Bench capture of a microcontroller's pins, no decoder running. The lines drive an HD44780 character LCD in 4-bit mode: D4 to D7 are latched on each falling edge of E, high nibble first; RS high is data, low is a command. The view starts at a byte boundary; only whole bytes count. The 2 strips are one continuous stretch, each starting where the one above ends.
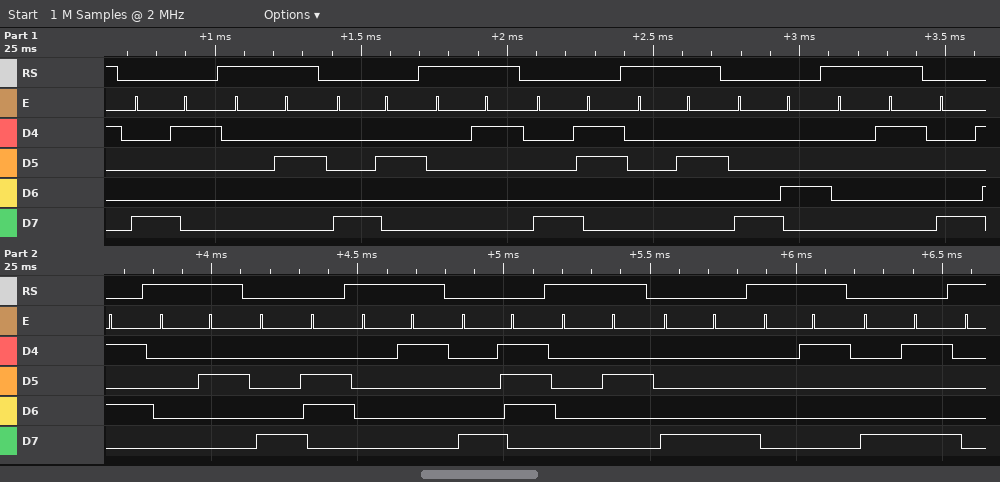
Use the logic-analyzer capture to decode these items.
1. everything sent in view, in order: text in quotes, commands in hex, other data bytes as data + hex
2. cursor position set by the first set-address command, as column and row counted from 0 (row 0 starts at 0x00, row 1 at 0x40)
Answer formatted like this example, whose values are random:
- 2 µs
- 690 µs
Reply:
- 0x81 data 02 0x82 data 01 0x83 data 02 0x84 data 01 0x85 data 02 0x86 data 01 0x87 data 02 0x88 data 01 0x89
- column 1, row 0
